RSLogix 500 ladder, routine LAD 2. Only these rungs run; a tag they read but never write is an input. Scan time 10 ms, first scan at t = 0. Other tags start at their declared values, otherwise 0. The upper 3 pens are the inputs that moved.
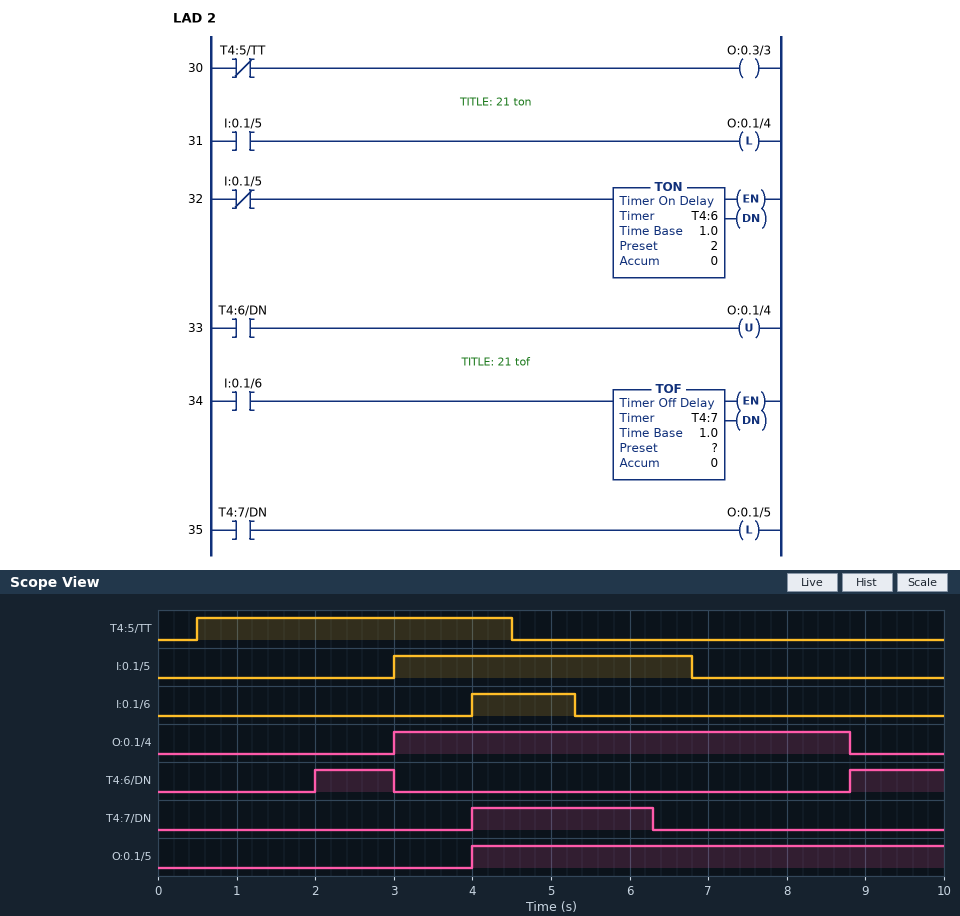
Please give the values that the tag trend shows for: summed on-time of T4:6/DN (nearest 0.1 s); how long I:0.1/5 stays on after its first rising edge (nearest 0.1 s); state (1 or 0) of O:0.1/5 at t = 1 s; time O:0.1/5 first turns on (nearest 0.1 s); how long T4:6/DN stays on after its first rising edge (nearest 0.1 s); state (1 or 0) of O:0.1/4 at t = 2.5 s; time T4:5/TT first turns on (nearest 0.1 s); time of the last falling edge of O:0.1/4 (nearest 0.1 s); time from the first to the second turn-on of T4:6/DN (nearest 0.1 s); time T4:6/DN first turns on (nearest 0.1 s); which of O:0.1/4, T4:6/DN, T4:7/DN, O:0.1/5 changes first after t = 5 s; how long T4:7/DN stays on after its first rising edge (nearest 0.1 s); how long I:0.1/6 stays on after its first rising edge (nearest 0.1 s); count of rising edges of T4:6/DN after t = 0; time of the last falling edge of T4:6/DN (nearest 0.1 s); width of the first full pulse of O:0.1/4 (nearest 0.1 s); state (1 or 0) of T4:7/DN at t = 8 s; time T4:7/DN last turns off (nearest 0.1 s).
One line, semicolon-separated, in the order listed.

2.2 s; 3.8 s; 0; 4.0 s; 1.0 s; 0; 0.5 s; 8.8 s; 6.8 s; 2.0 s; T4:7/DN; 2.3 s; 1.3 s; 2; 3.0 s; 5.8 s; 0; 6.3 s
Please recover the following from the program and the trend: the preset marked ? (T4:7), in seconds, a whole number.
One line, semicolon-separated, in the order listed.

1 s
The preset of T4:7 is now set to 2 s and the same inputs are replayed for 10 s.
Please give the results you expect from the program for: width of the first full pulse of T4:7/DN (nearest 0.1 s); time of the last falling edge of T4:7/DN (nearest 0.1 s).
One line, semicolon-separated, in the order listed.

3.3 s; 7.3 s
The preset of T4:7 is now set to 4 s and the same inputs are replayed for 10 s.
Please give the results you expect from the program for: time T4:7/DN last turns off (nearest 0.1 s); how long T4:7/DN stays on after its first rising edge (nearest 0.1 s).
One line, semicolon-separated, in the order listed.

9.3 s; 5.3 s
